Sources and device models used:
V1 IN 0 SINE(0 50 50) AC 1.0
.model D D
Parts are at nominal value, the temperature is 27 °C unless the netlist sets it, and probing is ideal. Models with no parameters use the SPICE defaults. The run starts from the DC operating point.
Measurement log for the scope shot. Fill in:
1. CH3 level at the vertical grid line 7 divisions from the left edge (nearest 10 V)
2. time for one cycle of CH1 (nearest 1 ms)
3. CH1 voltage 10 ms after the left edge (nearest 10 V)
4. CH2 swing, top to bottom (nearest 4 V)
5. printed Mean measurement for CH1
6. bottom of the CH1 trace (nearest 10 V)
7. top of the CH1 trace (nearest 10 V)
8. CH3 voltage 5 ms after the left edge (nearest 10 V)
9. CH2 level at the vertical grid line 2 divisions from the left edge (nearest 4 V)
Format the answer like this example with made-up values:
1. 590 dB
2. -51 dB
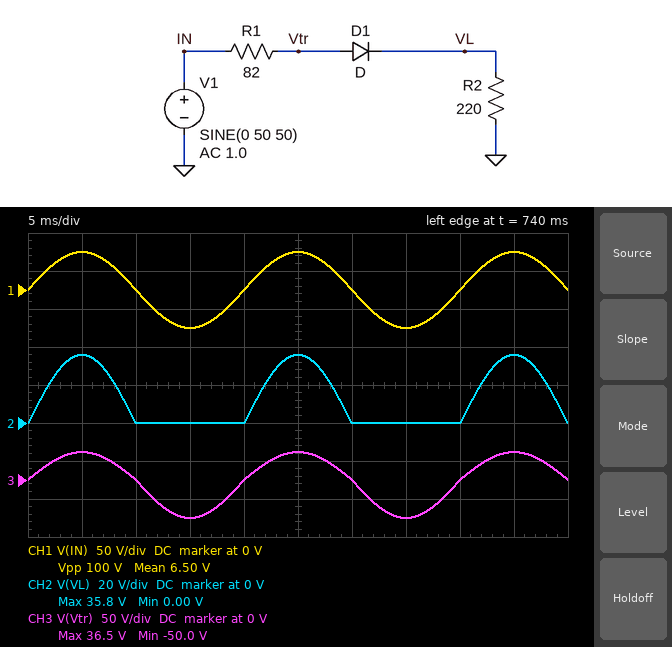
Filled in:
1. -50 V
2. 20 ms
3. 0 V
4. 36 V
5. 6.50 V
6. -50 V
7. 50 V
8. 40 V
9. 0 V
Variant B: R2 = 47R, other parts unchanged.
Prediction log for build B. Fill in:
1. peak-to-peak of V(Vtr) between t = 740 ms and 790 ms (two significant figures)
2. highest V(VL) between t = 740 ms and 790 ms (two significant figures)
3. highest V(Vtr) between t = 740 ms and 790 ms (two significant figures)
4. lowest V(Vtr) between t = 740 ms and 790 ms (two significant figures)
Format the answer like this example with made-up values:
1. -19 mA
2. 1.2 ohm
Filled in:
1. 69 V
2. 18 V
3. 19 V
4. -50 V
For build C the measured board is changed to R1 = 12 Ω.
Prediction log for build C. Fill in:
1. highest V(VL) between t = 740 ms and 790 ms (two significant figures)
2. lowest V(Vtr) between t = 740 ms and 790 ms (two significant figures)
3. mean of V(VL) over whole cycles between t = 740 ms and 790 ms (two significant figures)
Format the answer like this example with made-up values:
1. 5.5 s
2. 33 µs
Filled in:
1. 47 V
2. -50 V
3. 15 V
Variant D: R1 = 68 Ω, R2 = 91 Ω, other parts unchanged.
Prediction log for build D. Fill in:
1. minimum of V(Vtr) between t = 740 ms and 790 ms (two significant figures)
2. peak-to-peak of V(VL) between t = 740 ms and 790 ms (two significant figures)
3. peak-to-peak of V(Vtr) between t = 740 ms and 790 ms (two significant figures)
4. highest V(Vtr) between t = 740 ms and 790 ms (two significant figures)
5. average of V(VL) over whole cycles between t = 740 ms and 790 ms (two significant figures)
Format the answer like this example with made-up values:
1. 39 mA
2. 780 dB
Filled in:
1. -50 V
2. 28 V
3. 79 V
4. 29 V
5. 8.9 V
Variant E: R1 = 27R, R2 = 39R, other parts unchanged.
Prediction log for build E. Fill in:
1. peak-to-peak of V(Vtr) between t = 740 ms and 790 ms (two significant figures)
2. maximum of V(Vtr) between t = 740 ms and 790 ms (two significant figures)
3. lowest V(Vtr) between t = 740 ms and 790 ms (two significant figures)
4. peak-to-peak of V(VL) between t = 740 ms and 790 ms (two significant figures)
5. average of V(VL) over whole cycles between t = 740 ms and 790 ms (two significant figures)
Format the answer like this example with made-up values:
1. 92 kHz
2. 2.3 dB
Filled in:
1. 80 V
2. 30 V
3. -50 V
4. 29 V
5. 9.2 V
